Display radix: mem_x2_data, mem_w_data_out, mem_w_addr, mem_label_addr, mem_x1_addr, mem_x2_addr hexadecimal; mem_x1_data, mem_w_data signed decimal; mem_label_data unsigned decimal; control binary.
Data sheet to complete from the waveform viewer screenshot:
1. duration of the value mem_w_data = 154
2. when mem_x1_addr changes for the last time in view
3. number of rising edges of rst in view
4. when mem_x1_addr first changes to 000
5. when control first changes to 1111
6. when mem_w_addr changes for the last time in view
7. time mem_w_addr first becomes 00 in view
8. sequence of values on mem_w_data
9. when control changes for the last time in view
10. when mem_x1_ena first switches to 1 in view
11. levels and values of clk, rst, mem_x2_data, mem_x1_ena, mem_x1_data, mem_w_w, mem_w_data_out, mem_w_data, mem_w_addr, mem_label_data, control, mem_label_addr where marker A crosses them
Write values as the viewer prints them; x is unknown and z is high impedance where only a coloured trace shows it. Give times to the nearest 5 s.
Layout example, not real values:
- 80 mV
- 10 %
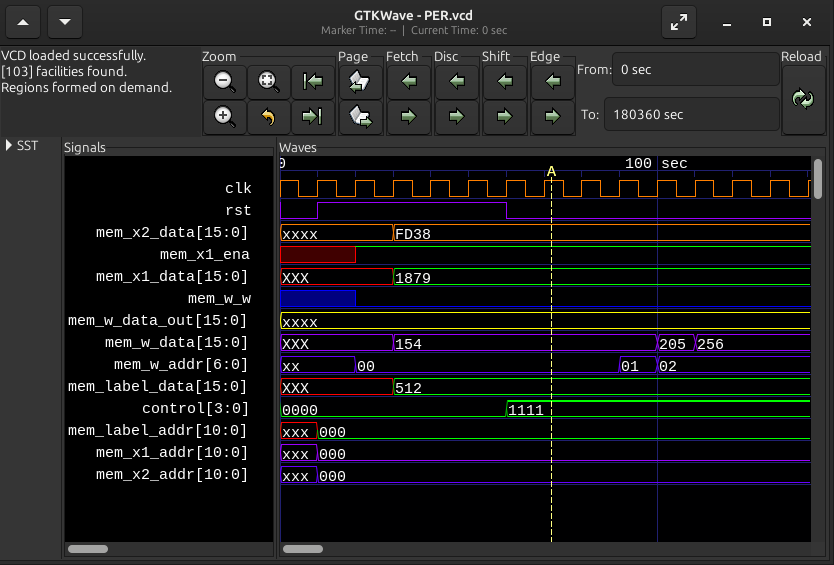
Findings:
- 70 s
- 10 s
- 1
- 10 s
- 60 s
- 100 s
- 20 s
- XXX, 154, 205, 256
- 60 s
- 20 s
- clk=1, rst=0, mem_x2_data=FD38, mem_x1_ena=1, mem_x1_data=1879, mem_w_w=0, mem_w_data_out=xxxx, mem_w_data=154, mem_w_addr=00, mem_label_data=512, control=1111, mem_label_addr=000
